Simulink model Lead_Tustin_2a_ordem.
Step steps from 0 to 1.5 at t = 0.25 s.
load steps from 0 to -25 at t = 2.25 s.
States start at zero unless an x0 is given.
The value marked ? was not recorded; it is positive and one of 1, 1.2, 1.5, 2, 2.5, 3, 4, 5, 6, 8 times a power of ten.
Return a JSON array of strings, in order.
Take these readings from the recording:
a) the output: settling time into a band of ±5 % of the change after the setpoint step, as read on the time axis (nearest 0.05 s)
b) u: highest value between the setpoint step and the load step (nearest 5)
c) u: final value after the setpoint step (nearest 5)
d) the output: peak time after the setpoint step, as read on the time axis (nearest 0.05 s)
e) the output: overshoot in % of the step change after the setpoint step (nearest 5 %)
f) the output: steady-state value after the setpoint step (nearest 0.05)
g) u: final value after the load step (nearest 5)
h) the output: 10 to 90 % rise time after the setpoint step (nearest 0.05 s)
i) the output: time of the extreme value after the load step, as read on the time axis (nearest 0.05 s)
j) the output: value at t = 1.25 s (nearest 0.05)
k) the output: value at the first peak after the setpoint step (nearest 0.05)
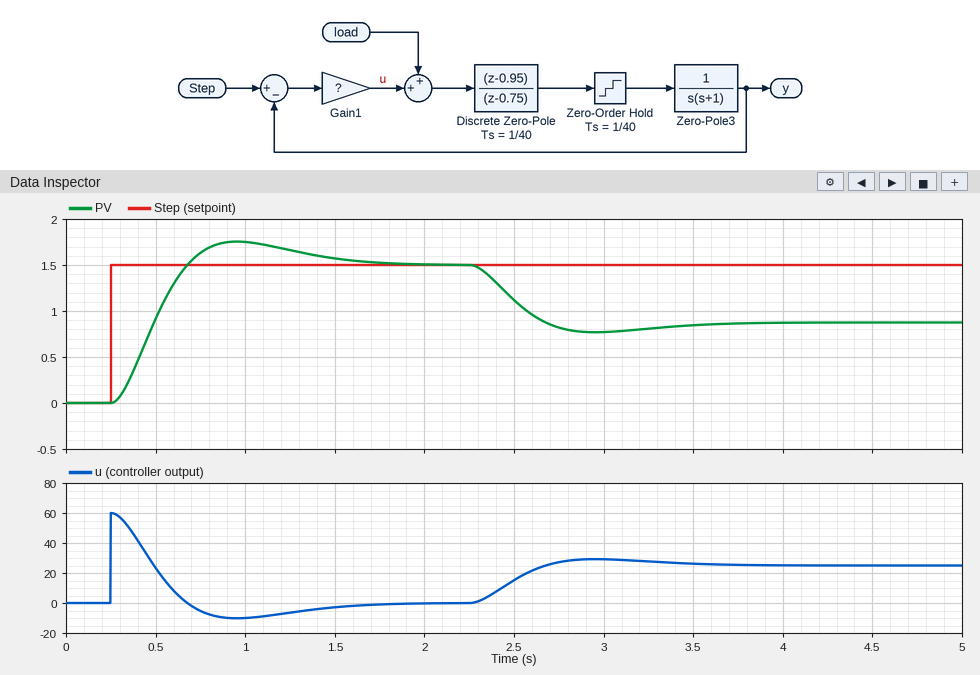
["1.50 s", "60", "0", "0.95 s", "15 %", "1.50", "25", "0.30 s", "2.95 s", "1.65", "1.75"]
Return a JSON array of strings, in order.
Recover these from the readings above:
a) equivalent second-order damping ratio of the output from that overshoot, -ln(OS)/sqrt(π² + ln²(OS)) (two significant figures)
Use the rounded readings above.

["0.52"]
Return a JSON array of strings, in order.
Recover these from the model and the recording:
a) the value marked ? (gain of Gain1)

["40"]
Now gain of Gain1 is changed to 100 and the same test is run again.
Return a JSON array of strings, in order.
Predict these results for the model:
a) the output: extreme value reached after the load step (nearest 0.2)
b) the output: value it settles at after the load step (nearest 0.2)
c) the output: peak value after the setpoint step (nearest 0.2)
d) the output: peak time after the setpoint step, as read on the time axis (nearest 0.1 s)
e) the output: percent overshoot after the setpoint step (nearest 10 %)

["1.2", "1.2", "2.0", "0.6 s", "30 %"]
